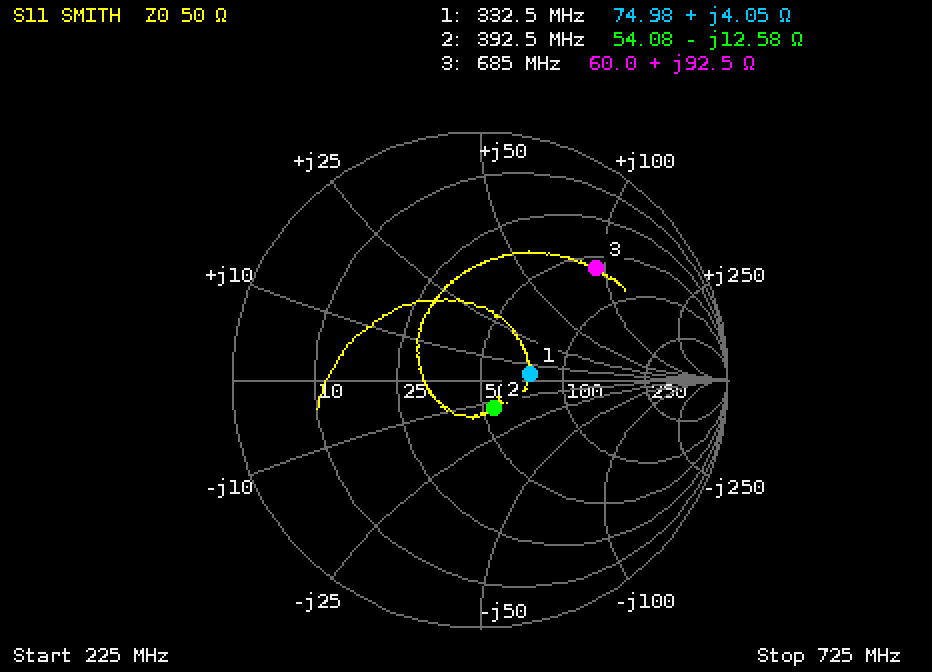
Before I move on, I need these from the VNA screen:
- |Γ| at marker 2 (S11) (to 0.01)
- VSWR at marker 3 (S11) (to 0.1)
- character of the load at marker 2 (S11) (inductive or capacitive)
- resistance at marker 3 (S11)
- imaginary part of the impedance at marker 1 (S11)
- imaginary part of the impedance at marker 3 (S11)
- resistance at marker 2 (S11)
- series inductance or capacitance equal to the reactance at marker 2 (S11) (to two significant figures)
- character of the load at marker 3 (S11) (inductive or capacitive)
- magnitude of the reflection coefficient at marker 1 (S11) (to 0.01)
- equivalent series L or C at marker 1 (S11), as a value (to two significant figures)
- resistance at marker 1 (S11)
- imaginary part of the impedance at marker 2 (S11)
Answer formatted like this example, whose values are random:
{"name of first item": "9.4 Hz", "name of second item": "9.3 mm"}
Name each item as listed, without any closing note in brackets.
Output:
{"|Γ| at marker 2 (S11)": "0.13", "VSWR at marker 3 (S11)": "4.7", "character of the load at marker 2 (S11)": "capacitive", "resistance at marker 3": "60.0 Ω", "imaginary part of the impedance at marker 1": "+4.05 Ω", "imaginary part of the impedance at marker 3": "+92.5 Ω", "resistance at marker 2": "54.08 Ω", "series inductance or capacitance equal to the reactance at marker 2 (S11)": "32 pF", "character of the load at marker 3 (S11)": "inductive", "magnitude of the reflection coefficient at marker 1 (S11)": "0.20", "equivalent series L or C at marker 1 (S11), as a value": "1.9 nH", "resistance at marker 1": "74.98 Ω", "imaginary part of the impedance at marker 2": "-12.58 Ω"}
